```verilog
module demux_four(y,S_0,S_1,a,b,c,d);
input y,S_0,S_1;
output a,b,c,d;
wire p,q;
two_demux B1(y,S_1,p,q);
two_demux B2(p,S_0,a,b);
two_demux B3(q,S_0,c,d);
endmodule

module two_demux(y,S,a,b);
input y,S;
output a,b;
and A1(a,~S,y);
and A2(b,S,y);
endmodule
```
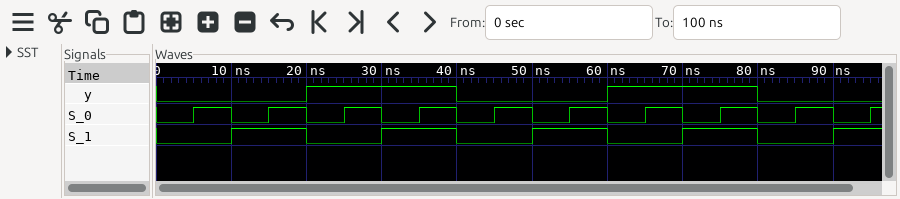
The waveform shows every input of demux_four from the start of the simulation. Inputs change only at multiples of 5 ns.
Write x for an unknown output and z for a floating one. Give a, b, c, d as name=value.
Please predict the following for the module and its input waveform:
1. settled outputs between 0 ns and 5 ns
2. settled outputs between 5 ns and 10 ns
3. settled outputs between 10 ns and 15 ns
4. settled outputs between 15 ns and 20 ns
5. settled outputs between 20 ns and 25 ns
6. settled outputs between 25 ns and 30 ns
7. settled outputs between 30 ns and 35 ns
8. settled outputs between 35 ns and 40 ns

a=0, b=0, c=0, d=0
a=0, b=0, c=0, d=0
a=0, b=0, c=0, d=0
a=0, b=0, c=0, d=0
a=1, b=0, c=0, d=0
a=0, b=1, c=0, d=0
a=0, b=0, c=1, d=0
a=0, b=0, c=0, d=1
